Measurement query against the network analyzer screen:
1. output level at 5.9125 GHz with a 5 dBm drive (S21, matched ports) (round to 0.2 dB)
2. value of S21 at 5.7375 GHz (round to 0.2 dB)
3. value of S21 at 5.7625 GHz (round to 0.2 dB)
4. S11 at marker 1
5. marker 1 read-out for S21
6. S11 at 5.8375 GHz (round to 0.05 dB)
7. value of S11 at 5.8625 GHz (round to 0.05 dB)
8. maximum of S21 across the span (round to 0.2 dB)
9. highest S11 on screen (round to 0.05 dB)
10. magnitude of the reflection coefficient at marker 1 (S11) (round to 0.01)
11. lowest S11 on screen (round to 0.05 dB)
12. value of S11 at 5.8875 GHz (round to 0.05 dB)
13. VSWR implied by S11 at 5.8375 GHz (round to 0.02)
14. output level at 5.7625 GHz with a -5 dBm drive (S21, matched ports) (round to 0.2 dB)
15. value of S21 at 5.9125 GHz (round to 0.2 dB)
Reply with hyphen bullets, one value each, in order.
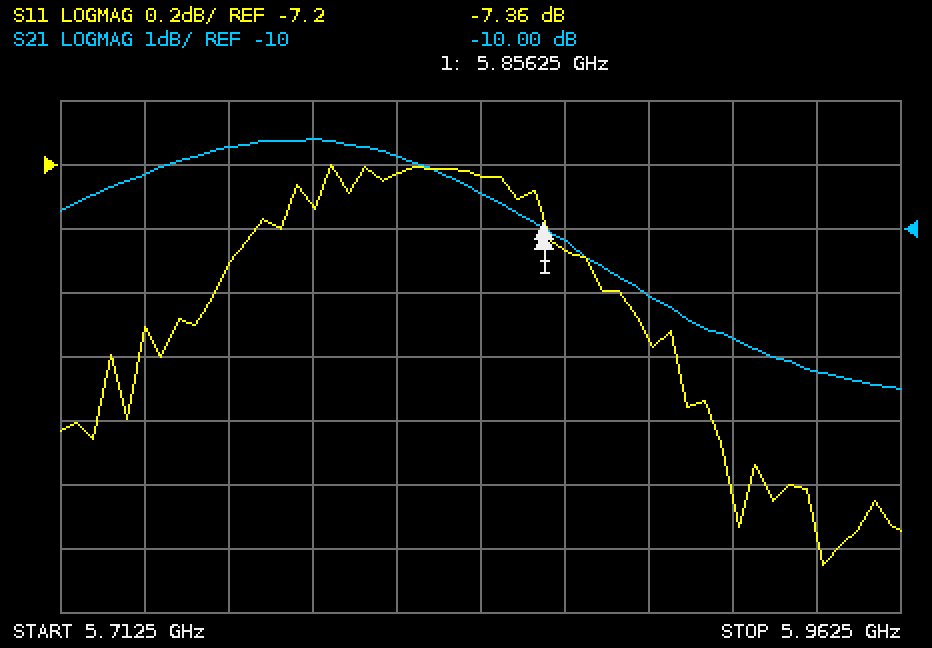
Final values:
- -6.8 dBm
- -9.2 dB
- -8.8 dB
- -7.36 dB
- -10.00 dB
- -7.25 dB
- -7.45 dB
- -8.6 dB
- -7.20 dB
- 0.43
- -8.45 dB
- -7.75 dB
- 2.54
- -13.8 dBm
- -11.8 dB
